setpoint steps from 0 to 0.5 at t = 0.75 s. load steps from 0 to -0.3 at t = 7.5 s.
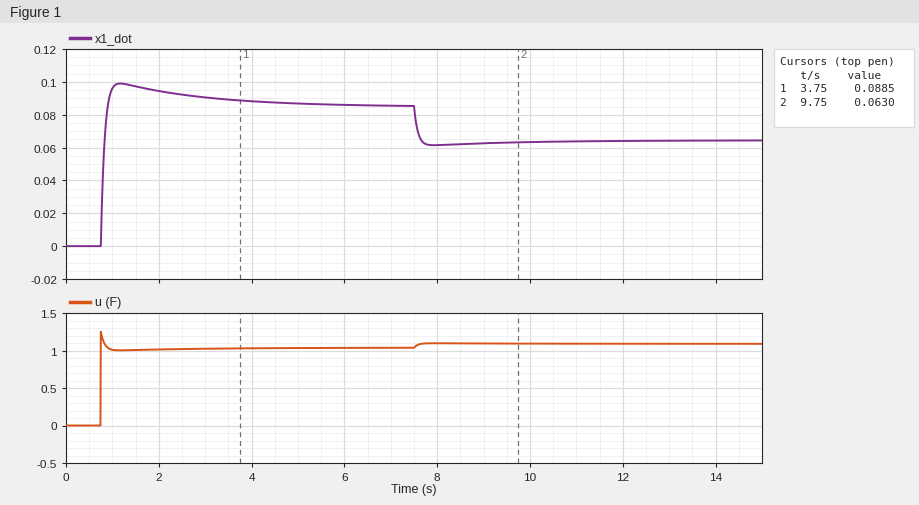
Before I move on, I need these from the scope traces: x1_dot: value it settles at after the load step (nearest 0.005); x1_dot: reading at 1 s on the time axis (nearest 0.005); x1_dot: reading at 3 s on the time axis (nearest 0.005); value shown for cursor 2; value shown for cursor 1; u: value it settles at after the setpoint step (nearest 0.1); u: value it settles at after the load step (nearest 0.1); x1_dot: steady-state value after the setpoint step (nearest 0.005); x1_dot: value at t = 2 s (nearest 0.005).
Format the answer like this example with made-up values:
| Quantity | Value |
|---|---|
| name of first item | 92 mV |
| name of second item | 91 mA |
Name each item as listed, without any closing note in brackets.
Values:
| Quantity | Value |
|---|---|
| x1_dot: value it settles at after the load step | 0.065 |
| x1_dot: reading at 1 s on the time axis | 0.095 |
| x1_dot: reading at 3 s on the time axis | 0.090 |
| value shown for cursor 2 | 0.0630 |
| value shown for cursor 1 | 0.0885 |
| u: value it settles at after the setpoint step | 1.0 |
| u: value it settles at after the load step | 1.1 |
| x1_dot: steady-state value after the setpoint step | 0.085 |
| x1_dot: value at t = 2 s | 0.095 |
